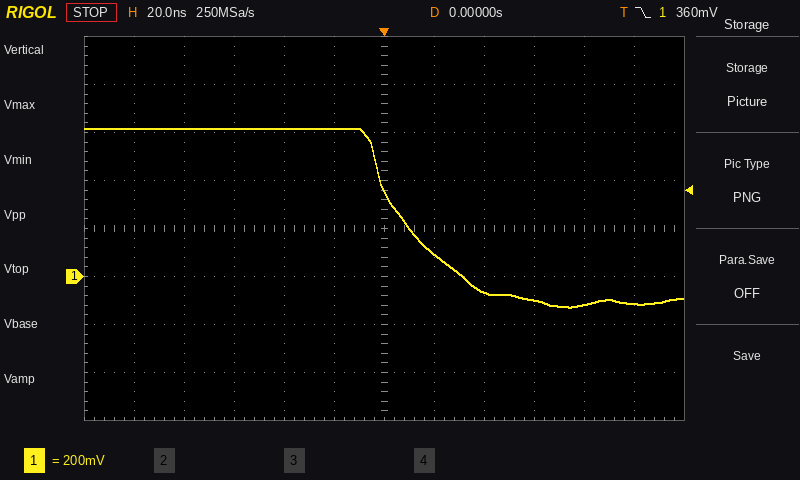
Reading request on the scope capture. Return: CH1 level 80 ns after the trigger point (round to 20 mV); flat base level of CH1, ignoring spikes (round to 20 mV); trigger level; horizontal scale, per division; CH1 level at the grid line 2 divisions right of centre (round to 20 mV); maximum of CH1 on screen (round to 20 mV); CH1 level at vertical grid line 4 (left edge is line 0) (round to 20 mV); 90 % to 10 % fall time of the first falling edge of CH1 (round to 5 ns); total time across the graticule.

-120 mV
-100 mV
360 mV
20 ns
-60 mV
620 mV
620 mV
40 ns
240 ns
